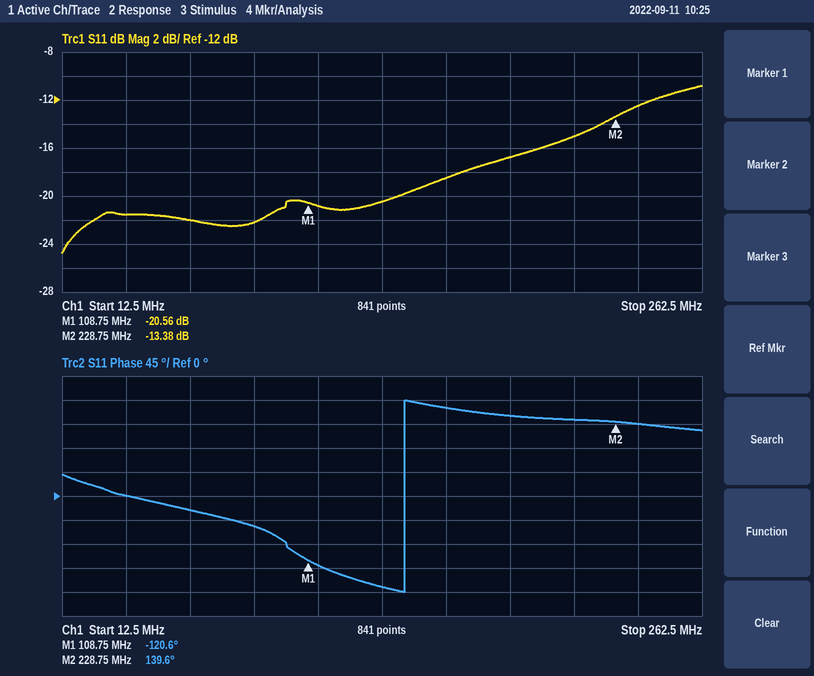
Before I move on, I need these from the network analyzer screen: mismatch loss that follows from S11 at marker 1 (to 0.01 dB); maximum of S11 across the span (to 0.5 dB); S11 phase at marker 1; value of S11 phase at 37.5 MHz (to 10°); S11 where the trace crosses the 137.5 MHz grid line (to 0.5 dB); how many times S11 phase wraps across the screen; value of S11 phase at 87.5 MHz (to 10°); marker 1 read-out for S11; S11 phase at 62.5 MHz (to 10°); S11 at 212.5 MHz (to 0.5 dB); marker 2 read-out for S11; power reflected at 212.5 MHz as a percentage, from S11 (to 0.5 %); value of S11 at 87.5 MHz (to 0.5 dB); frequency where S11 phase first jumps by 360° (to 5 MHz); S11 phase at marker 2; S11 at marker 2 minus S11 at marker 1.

0.04 dB
-11.0 dB
-120.6°
0°
-20.5 dB
1
-60°
-20.56 dB
-30°
-15.0 dB
-13.38 dB
3.0 %
-22.0 dB
145 MHz
139.6°
7.18 dB
